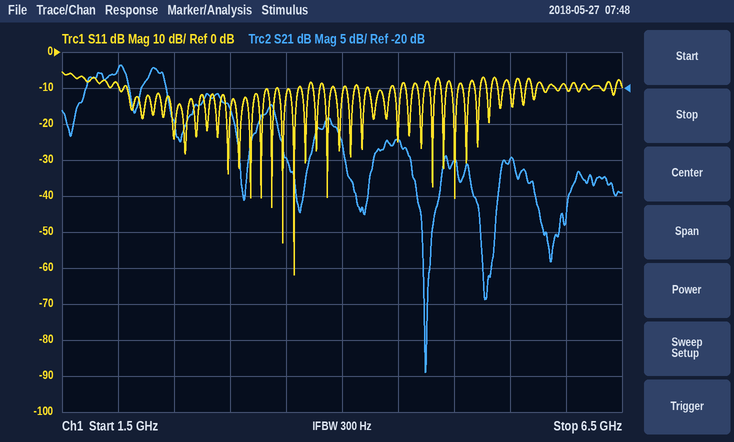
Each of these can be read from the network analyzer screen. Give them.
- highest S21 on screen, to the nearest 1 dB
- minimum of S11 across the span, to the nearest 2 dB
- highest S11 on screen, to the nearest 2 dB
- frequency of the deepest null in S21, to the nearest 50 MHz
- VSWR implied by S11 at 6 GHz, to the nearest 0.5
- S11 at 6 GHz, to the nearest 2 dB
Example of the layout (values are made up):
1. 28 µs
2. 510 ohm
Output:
1. -17 dB
2. -62 dB
3. -6 dB
4. 4.75 GHz
5. 2.0
6. -10 dB
